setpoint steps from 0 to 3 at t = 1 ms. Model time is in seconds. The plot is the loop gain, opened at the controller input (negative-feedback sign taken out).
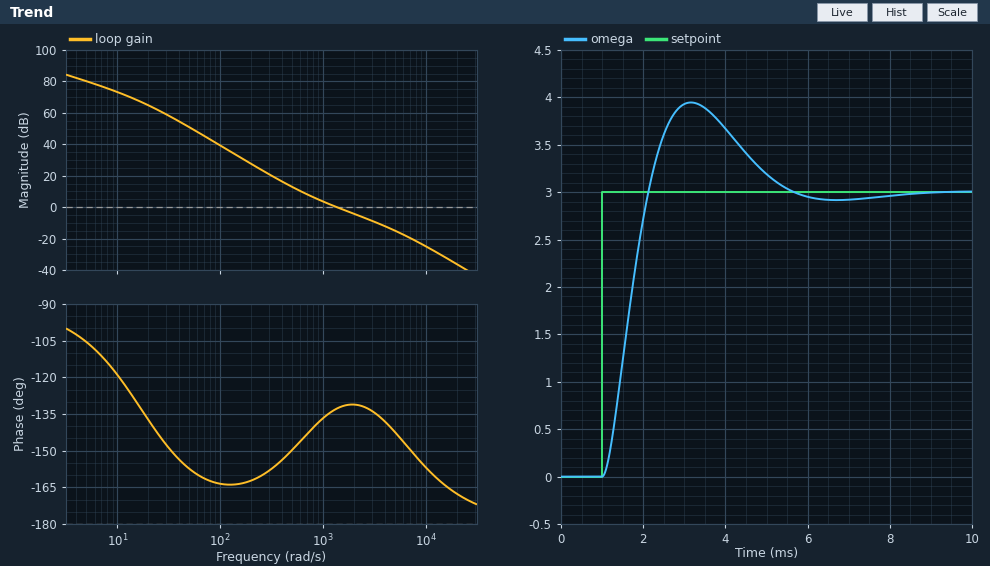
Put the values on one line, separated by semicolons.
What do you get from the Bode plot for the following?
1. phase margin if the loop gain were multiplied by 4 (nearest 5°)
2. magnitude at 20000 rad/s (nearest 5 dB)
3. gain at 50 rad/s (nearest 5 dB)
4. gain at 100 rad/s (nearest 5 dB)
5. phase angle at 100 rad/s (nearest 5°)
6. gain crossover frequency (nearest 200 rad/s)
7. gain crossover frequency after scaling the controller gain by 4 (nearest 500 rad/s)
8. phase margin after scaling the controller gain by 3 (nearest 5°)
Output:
40°; -35 dB; 50 dB; 40 dB; -165°; 1400 rad/s; 4000 rad/s; 45°
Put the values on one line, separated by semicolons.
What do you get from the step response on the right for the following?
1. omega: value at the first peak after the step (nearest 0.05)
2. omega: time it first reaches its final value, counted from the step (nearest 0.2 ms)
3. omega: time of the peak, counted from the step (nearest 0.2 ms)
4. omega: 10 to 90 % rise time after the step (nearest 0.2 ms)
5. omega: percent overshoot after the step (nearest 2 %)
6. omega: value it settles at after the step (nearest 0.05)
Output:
3.95; 1.2 ms; 2.2 ms; 0.8 ms; 32 %; 3.00
